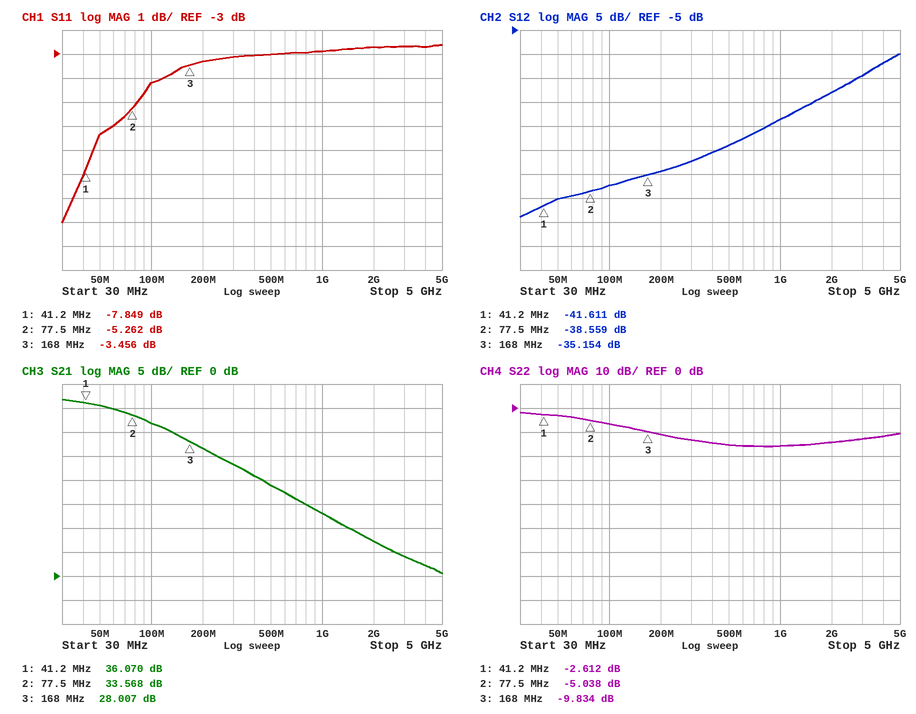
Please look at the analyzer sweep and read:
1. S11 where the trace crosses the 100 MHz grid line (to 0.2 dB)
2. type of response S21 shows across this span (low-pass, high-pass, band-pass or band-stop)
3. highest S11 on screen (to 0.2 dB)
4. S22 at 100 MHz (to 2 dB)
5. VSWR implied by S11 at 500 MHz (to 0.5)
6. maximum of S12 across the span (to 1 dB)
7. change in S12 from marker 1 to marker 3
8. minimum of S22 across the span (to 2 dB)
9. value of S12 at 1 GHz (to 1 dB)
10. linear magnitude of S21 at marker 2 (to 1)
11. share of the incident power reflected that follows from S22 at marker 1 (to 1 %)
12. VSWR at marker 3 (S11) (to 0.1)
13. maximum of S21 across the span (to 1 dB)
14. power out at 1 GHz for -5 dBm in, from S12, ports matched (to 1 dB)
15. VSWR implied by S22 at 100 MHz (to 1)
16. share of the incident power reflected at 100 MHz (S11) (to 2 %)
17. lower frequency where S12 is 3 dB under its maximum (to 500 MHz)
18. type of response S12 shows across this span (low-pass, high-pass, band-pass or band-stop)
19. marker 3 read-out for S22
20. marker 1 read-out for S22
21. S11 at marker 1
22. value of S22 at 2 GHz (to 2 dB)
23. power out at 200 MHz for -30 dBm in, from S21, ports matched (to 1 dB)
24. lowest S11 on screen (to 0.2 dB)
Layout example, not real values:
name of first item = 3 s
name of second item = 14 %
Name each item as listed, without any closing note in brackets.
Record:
S11 where the trace crosses the 100 MHz grid line = -4.2 dB
type of response S21 shows across this span = low-pass
highest S11 on screen = -2.6 dB
S22 at 100 MHz = -6 dB
VSWR implied by S11 at 500 MHz = 6.0
maximum of S12 across the span = -10 dB
change in S12 from marker 1 to marker 3 = 6.457 dB
minimum of S22 across the span = -16 dB
value of S12 at 1 GHz = -24 dB
linear magnitude of S21 at marker 2 = 48
share of the incident power reflected that follows from S22 at marker 1 = 55 %
VSWR at marker 3 (S11) = 5.1
maximum of S21 across the span = 37 dB
power out at 1 GHz for -5 dBm in, from S12, ports matched = -29 dBm
VSWR implied by S22 at 100 MHz = 3
share of the incident power reflected at 100 MHz (S11) = 38 %
lower frequency where S12 is 3 dB under its maximum = 3.5 GHz
type of response S12 shows across this span = high-pass
marker 3 read-out for S22 = -9.834 dB
marker 1 read-out for S22 = -2.612 dB
S11 at marker 1 = -7.849 dB
value of S22 at 2 GHz = -14 dB
power out at 200 MHz for -30 dBm in, from S21, ports matched = -3 dBm
lowest S11 on screen = -10.0 dB
